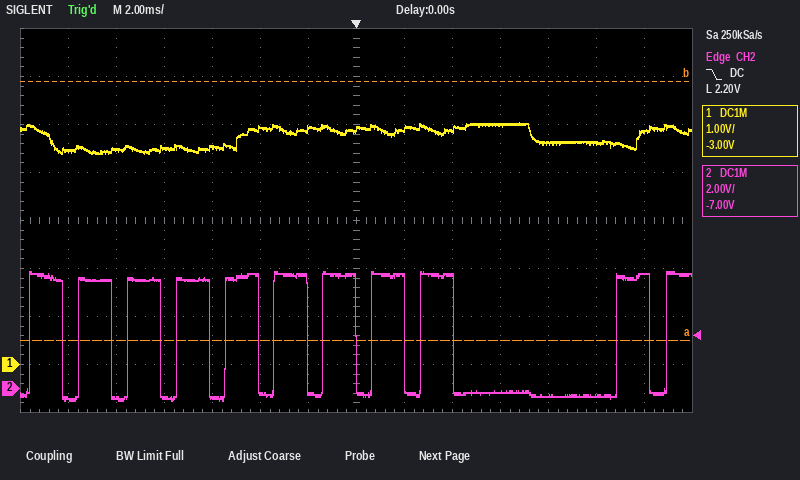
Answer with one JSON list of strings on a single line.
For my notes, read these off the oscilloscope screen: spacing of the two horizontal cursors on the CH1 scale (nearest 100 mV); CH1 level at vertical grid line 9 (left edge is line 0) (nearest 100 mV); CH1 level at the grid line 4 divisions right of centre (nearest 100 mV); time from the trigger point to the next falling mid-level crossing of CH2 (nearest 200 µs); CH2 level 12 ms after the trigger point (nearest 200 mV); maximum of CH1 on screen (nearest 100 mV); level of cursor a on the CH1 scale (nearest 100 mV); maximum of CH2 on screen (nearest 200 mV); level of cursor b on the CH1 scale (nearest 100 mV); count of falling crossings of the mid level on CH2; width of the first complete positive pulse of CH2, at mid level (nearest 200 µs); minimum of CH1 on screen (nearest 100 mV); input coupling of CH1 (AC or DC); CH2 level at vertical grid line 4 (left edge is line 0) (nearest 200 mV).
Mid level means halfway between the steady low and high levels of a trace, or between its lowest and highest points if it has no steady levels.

["5.4 V", "4.9 V", "4.6 V", "2.0 ms", "4.8 V", "5.0 V", "500 mV", "4.8 V", "5.9 V", "10", "1.4 ms", "4.4 V", "DC", "-400 mV"]
